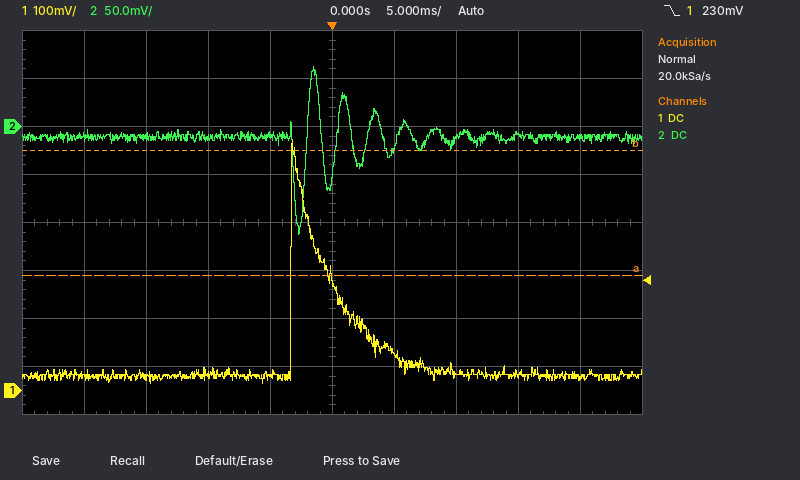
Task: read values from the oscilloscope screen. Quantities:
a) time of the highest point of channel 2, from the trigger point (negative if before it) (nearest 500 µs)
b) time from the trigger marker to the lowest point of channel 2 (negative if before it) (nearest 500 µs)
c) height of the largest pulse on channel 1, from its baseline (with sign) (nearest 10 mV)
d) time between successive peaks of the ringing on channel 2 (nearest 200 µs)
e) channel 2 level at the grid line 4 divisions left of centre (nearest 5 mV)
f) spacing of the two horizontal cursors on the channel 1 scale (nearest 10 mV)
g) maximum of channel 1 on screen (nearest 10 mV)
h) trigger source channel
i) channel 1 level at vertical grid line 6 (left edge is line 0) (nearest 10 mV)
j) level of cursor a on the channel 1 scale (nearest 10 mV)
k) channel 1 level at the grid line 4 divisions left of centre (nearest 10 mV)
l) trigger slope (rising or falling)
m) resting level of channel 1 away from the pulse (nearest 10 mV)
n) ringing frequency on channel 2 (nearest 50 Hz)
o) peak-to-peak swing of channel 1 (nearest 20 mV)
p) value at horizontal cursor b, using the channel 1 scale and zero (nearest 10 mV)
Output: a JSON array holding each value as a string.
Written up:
["-1.5 ms", "-2.5 ms", "+490 mV", "2.4 ms", "-10 mV", "260 mV", "520 mV", "channel 1", "80 mV", "240 mV", "30 mV", "falling", "30 mV", "400 Hz", "500 mV", "500 mV"]
